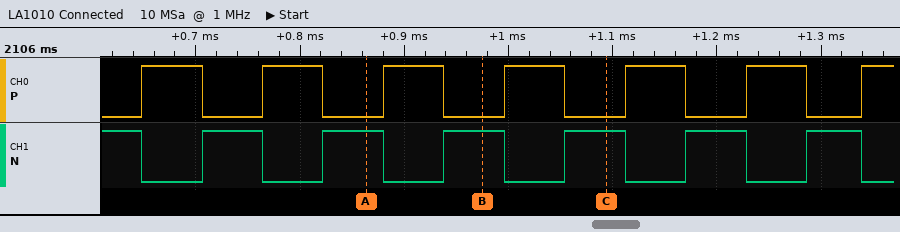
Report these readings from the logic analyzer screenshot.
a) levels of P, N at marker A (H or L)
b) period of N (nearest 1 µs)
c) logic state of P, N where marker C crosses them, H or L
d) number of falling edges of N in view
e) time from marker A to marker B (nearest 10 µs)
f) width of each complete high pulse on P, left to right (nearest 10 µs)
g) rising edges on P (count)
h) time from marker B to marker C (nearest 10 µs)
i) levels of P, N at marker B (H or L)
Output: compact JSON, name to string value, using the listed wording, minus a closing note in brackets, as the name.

{"levels of P, N at marker A": "P=L, N=H", "period of N": "116 µs", "logic state of P, N where marker C crosses them, H or L": "P=L, N=H", "number of falling edges of N in view": "7", "time from marker A to marker B": "110 µs", "width of each complete high pulse on P, left to right": "60 µs, 60 µs, 60 µs, 60 µs, 60 µs, 60 µs", "rising edges on P": "7", "time from marker B to marker C": "120 µs", "levels of P, N at marker B": "P=L, N=H"}
